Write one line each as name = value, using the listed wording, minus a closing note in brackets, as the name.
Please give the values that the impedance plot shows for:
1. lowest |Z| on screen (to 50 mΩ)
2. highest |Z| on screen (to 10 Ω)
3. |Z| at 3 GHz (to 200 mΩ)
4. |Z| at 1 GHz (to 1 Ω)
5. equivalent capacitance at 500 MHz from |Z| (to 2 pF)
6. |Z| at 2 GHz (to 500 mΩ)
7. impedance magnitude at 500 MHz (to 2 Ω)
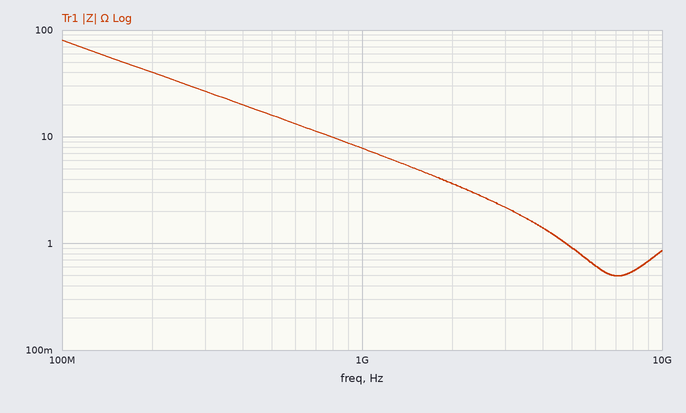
lowest |Z| on screen = 500 mΩ
highest |Z| on screen = 80 Ω
|Z| at 3 GHz = 2.2 Ω
|Z| at 1 GHz = 8 Ω
equivalent capacitance at 500 MHz from |Z| = 20 pF
|Z| at 2 GHz = 3.5 Ω
impedance magnitude at 500 MHz = 16 Ω
